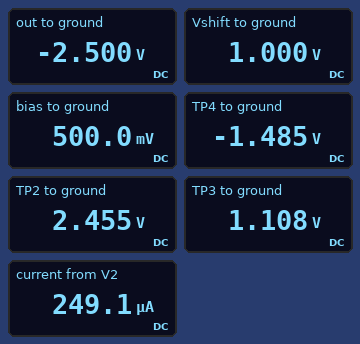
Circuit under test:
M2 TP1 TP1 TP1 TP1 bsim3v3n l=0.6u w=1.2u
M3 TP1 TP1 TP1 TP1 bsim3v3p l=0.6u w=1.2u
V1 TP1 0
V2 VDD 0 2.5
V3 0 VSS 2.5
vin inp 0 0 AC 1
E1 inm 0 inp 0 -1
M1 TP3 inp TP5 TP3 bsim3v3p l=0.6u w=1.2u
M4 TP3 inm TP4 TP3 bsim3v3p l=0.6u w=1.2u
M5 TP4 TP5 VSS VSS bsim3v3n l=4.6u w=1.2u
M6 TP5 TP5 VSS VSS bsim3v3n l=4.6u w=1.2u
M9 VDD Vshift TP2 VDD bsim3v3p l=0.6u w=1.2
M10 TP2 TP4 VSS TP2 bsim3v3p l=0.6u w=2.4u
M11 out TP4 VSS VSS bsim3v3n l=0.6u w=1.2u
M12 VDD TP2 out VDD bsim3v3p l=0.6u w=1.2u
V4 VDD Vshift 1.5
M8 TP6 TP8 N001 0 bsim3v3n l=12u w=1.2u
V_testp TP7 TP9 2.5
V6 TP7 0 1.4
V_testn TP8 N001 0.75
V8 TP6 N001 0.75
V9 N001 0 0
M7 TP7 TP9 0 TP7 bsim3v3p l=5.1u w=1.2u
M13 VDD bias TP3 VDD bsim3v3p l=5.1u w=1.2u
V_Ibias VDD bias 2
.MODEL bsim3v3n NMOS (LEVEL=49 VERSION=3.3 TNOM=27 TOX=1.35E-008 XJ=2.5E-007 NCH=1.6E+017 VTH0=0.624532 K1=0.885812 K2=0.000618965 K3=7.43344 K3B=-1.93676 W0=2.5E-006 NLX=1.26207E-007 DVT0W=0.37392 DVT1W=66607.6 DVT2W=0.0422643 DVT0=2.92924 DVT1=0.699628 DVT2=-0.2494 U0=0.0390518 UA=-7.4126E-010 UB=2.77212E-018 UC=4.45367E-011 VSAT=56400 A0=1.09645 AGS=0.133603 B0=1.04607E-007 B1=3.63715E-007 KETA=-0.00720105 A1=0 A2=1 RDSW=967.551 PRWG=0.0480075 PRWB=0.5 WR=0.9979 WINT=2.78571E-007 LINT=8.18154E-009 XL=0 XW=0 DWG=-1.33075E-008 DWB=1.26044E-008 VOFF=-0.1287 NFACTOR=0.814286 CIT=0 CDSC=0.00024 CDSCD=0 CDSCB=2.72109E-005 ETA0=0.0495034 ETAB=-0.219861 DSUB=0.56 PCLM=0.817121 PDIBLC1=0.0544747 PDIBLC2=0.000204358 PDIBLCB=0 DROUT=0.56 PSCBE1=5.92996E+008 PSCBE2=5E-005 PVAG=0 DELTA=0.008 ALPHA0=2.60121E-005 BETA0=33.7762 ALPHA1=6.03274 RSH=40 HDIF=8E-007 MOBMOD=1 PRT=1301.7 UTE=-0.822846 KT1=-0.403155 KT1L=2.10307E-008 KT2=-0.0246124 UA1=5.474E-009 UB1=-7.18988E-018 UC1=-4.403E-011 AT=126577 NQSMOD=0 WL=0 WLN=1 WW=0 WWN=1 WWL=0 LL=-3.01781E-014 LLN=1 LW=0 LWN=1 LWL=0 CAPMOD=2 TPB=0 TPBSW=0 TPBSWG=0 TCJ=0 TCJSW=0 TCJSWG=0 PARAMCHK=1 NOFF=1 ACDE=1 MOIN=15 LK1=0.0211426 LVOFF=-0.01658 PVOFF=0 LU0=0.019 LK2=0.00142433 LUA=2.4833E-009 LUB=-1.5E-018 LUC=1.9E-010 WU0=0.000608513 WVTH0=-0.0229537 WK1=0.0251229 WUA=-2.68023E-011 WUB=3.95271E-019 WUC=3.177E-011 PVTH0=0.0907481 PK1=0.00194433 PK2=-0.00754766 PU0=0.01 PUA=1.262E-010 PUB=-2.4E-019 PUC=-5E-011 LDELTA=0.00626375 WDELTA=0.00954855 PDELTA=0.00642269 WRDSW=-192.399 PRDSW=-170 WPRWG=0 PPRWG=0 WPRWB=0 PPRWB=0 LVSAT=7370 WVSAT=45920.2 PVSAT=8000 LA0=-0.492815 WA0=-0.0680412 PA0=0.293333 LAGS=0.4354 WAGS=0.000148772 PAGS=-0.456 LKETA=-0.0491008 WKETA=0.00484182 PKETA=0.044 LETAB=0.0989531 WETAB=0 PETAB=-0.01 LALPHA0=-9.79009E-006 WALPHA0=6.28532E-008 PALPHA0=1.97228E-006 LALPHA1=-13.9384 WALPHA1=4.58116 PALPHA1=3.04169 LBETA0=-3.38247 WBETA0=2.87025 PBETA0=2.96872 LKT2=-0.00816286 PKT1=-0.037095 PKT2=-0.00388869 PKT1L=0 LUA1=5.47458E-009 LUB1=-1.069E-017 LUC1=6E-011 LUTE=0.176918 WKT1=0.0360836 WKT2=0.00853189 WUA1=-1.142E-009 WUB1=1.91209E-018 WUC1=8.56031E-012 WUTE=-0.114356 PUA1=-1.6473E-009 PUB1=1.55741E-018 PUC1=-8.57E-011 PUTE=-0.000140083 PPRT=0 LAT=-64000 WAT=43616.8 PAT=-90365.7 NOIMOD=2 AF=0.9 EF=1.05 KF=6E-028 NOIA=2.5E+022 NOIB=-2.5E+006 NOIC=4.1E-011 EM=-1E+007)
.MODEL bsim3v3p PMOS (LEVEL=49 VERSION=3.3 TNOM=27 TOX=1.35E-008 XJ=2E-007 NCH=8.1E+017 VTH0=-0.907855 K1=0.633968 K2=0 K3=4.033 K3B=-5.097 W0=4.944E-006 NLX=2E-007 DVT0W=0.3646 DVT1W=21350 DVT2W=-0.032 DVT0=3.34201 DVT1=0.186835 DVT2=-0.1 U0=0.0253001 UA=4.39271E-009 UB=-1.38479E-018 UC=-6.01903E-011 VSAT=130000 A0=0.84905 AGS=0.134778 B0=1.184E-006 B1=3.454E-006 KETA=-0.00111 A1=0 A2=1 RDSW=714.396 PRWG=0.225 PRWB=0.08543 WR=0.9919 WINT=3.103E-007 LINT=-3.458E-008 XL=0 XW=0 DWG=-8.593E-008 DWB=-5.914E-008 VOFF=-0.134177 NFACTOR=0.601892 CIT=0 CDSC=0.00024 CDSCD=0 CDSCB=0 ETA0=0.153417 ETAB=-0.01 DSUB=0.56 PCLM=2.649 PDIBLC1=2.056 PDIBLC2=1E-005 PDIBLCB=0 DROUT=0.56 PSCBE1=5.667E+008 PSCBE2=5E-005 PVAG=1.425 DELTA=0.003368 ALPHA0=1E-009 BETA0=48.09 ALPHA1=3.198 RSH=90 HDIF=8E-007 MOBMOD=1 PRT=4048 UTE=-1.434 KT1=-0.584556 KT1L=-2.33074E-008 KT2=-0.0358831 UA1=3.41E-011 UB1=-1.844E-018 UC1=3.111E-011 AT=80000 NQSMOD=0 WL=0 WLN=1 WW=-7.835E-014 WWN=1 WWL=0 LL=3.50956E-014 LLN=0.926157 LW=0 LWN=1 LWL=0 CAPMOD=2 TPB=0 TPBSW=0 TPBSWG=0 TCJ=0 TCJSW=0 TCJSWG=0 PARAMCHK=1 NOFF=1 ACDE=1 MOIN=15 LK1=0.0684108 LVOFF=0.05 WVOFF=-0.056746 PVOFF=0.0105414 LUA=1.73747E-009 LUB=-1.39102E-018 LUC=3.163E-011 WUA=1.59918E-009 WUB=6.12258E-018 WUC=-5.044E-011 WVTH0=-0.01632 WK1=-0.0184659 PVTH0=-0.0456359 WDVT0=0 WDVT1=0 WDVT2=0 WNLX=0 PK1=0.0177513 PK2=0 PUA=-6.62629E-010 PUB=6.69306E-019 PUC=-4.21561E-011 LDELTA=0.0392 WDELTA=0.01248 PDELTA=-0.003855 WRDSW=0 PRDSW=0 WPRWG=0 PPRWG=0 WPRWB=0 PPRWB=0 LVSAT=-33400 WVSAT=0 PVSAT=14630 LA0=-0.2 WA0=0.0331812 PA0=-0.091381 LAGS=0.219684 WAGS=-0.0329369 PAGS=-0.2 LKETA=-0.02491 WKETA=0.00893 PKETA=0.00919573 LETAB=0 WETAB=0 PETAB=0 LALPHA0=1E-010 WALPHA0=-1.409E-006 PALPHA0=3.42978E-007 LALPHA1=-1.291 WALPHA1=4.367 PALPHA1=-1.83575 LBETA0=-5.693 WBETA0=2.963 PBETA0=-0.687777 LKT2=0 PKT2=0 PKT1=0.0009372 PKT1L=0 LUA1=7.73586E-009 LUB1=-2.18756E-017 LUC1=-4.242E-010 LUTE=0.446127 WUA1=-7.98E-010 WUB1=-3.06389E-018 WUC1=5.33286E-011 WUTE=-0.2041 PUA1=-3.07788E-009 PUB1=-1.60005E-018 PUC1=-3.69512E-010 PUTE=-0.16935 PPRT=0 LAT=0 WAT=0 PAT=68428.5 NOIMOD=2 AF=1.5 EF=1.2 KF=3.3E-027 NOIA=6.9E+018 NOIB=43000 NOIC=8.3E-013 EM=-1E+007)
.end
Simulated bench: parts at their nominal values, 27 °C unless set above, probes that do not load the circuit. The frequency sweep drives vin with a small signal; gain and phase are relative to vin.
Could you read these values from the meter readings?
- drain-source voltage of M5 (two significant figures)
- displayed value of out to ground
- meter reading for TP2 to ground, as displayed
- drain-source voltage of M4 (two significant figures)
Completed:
1.0 V
-2.500 V
2.455 V
2.6 V
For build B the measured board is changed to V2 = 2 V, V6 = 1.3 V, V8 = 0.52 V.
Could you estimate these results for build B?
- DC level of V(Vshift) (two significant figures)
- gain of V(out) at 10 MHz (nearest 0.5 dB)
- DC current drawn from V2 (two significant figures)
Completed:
500 mV
-27.0 dB
190 µA
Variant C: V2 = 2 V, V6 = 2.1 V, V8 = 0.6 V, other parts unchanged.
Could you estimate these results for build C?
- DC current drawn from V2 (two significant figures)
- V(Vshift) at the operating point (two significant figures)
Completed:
190 µA
500 mV
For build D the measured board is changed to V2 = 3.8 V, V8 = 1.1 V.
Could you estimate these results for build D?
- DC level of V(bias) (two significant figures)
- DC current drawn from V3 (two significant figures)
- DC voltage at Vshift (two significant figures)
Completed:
1.8 V
430 µA
2.3 V
